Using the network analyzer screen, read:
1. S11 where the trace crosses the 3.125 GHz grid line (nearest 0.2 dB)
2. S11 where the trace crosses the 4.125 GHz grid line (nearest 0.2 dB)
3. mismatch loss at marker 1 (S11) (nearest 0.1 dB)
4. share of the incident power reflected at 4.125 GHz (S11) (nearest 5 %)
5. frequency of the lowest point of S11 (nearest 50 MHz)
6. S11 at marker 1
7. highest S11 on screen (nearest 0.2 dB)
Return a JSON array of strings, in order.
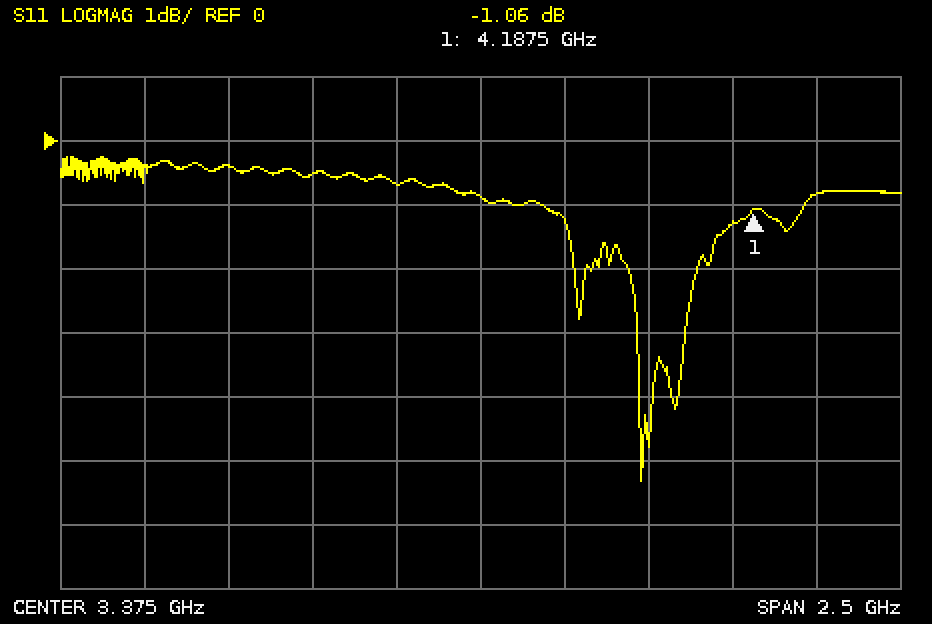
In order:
["-0.6 dB", "-1.2 dB", "6.6 dB", "75 %", "3.85 GHz", "-1.06 dB", "-0.2 dB"]
